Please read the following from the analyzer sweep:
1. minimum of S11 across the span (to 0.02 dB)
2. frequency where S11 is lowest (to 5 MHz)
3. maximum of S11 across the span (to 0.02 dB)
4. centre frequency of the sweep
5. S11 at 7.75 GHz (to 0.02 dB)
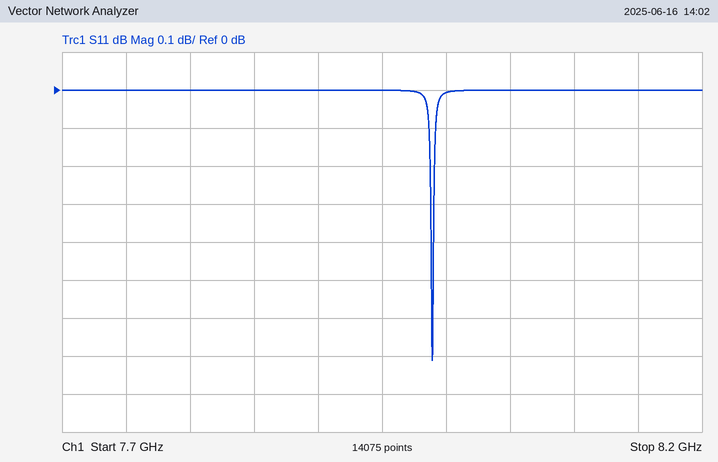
-0.72 dB
7.990 GHz
0.00 dB
7.95 GHz
0.00 dB
